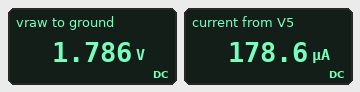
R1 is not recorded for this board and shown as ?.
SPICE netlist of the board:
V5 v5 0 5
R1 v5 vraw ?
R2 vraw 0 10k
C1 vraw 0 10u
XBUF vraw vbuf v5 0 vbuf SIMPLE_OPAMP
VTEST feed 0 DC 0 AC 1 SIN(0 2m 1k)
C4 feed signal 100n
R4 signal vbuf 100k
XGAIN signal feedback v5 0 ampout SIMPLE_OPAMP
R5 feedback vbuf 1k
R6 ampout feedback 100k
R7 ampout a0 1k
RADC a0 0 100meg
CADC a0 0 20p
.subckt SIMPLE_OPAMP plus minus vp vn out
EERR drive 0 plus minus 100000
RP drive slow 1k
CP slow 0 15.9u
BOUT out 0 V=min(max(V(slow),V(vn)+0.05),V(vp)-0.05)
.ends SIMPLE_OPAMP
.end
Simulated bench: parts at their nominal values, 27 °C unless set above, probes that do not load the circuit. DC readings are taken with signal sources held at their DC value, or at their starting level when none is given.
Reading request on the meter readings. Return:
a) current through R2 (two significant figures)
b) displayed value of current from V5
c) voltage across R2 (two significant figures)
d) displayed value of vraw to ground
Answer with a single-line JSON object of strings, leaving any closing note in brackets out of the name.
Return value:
{"current through R2": "180 µA", "displayed value of current from V5": "178.6 µA", "voltage across R2": "1.8 V", "displayed value of vraw to ground": "1.786 V"}
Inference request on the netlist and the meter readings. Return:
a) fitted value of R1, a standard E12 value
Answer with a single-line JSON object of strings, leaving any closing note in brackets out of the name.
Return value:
{"fitted value of R1, a standard E12 value": "18 kΩ"}
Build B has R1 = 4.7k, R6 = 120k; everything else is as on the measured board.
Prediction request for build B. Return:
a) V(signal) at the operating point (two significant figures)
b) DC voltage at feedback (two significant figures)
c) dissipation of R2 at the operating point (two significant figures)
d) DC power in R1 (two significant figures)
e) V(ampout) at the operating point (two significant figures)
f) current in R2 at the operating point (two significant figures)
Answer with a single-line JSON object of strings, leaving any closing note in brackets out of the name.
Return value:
{"V(signal) at the operating point": "55 mV", "DC voltage at feedback": "4.9 V", "dissipation of R2 at the operating point": "480 nW", "DC power in R1": "5.2 mW", "V(ampout) at the operating point": "50 mV", "current in R2 at the operating point": "6.9 µA"}
